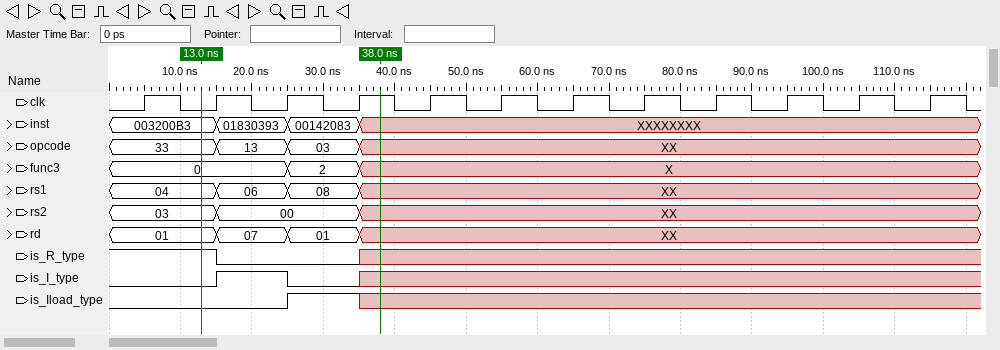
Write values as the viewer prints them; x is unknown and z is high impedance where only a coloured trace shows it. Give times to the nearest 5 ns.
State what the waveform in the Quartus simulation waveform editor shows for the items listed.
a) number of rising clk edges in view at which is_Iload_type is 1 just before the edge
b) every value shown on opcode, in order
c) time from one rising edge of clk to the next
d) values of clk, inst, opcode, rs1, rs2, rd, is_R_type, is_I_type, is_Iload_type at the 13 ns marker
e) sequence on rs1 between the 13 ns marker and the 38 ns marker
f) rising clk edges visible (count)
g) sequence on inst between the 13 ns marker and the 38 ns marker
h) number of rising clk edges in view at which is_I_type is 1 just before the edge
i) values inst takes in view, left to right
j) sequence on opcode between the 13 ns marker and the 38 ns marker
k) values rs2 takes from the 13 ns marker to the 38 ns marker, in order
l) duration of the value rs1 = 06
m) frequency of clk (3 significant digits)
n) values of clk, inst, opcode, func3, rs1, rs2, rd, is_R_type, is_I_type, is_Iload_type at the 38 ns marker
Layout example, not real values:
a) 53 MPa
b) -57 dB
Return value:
a) 1
b) 33, 13, 03, XX
c) 10 ns
d) clk=0, inst=003200B3, opcode=33, rs1=04, rs2=03, rd=01, is_R_type=1, is_I_type=0, is_Iload_type=0
e) 04, 06, 08, XX
f) 12
g) 003200B3, 01830393, 00142083, XXXXXXXX
h) 1
i) 003200B3, 01830393, 00142083, XXXXXXXX
j) 33, 13, 03, XX
k) 03, 00, XX
l) 10 ns
m) 100 MHz
n) clk=1, inst=XXXXXXXX, opcode=XX, func3=X, rs1=XX, rs2=XX, rd=XX, is_R_type=x, is_I_type=x, is_Iload_type=x
